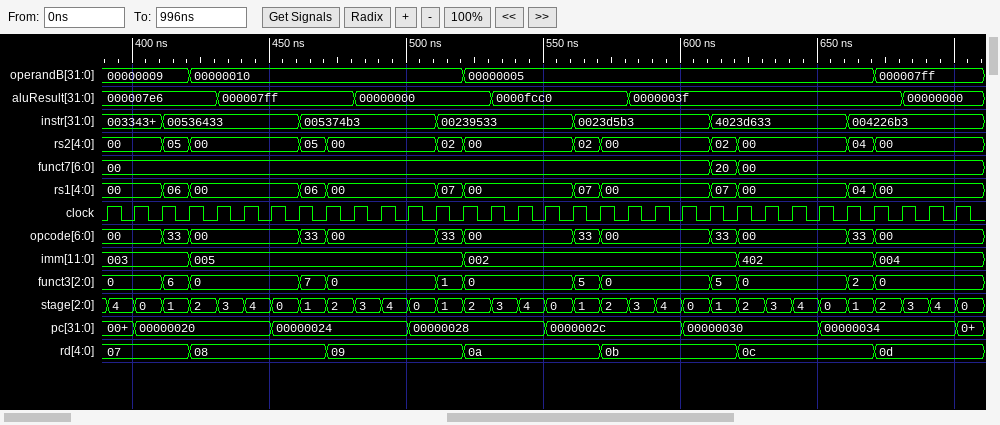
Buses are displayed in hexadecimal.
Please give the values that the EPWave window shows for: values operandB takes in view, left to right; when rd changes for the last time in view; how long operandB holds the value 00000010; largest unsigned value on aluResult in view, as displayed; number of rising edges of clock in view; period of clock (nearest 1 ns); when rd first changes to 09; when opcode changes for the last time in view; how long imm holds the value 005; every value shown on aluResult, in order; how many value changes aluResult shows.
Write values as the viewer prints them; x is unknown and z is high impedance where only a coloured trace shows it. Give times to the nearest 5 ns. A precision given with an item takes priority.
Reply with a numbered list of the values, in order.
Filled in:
1. 00000009, 00000010, 00000005, 000007ff
2. 670 ns
3. 100 ns
4. 0000fcc0
5. 32
6. 10 ns
7. 470 ns
8. 670 ns
9. 100 ns
10. 000007e6, 000007ff, 00000000, 0000fcc0, 0000003f, 00000000
11. 5
